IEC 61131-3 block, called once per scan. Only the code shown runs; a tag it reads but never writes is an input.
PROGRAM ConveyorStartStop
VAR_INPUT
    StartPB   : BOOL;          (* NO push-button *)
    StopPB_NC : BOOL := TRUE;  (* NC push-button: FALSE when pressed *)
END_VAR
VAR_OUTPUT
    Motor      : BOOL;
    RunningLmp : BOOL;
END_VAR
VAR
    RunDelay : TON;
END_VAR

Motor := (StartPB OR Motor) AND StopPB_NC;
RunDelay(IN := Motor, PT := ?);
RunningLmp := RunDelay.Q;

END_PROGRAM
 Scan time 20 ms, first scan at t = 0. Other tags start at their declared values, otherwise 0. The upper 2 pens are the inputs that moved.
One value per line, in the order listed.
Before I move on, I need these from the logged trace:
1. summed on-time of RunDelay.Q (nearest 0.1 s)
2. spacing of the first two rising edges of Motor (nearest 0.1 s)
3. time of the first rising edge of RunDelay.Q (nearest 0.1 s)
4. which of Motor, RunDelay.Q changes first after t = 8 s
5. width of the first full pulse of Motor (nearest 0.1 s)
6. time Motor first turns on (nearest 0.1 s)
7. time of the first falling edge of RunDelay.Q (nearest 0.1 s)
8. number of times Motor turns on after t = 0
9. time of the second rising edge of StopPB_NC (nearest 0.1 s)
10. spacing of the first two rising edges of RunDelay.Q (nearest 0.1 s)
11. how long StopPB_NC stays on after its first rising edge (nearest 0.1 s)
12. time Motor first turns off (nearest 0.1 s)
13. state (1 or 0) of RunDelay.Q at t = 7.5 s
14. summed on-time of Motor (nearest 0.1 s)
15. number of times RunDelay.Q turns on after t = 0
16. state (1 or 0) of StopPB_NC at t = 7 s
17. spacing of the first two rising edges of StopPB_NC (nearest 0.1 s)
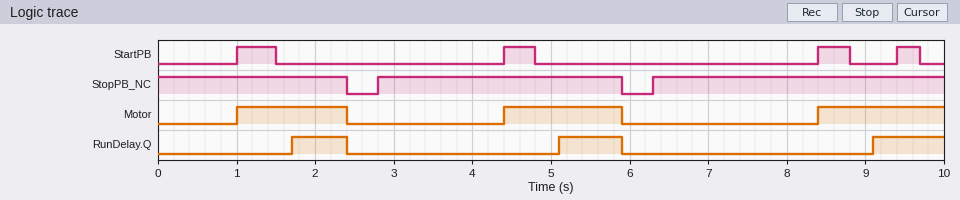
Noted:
2.4 s
3.4 s
1.7 s
Motor
1.4 s
1.0 s
2.4 s
3
6.3 s
3.4 s
3.1 s
2.4 s
0
4.5 s
3
1
3.5 s
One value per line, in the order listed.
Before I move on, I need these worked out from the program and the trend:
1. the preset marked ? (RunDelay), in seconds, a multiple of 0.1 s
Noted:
0.7 s
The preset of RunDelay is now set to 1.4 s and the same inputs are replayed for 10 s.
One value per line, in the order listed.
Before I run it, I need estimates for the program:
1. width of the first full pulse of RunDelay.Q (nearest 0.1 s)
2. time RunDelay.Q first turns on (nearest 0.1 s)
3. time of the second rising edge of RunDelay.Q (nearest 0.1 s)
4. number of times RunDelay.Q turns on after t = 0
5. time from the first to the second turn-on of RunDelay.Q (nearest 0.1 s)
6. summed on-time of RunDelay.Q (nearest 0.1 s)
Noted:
0.1 s
5.8 s
9.8 s
2
4.0 s
0.3 s
